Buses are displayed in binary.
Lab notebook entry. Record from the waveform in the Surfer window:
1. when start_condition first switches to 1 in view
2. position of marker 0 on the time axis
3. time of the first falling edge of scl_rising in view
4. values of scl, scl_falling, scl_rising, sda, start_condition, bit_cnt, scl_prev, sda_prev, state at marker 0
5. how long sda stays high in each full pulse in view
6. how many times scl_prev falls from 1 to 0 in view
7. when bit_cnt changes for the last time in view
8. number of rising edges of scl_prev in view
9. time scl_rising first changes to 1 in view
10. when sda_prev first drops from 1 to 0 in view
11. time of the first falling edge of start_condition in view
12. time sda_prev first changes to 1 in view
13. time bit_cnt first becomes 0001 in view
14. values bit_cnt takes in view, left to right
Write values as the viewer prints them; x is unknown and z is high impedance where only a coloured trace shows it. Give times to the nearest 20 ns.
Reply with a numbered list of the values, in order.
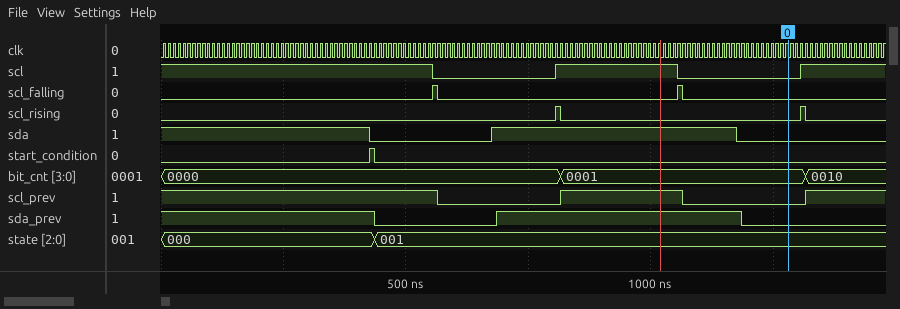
1. 420 ns
2. 1280 ns
3. 820 ns
4. scl=0, scl_falling=0, scl_rising=0, sda=0, start_condition=0, bit_cnt=0001, scl_prev=0, sda_prev=0, state=001
5. 500 ns
6. 2
7. 1320 ns
8. 2
9. 800 ns
10. 440 ns
11. 440 ns
12. 680 ns
13. 820 ns
14. 0000, 0001, 0010
